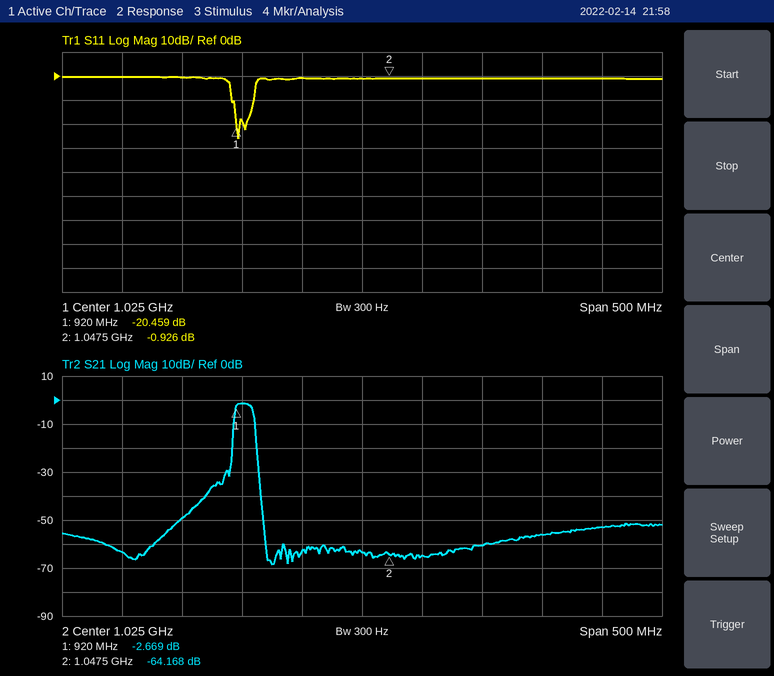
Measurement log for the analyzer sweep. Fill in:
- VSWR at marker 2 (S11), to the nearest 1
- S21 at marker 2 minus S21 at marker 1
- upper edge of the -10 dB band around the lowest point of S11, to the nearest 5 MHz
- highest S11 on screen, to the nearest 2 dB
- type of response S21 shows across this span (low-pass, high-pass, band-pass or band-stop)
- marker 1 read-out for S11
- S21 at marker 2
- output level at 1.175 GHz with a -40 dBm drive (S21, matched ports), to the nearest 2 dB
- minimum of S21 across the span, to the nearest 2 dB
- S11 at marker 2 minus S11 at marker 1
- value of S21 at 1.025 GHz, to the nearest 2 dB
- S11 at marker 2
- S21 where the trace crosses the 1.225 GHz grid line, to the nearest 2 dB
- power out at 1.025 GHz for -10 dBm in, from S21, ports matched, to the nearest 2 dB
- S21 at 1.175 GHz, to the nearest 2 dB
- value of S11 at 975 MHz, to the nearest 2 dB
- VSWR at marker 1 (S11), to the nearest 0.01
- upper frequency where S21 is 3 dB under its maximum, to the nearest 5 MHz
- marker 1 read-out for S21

19
-61.499 dB
935 MHz
0 dB
band-pass
-20.459 dB
-64.168 dB
-96 dBm
-68 dB
19.533 dB
-64 dB
-0.926 dB
-52 dB
-74 dBm
-56 dB
0 dB
1.21
935 MHz
-2.669 dB
